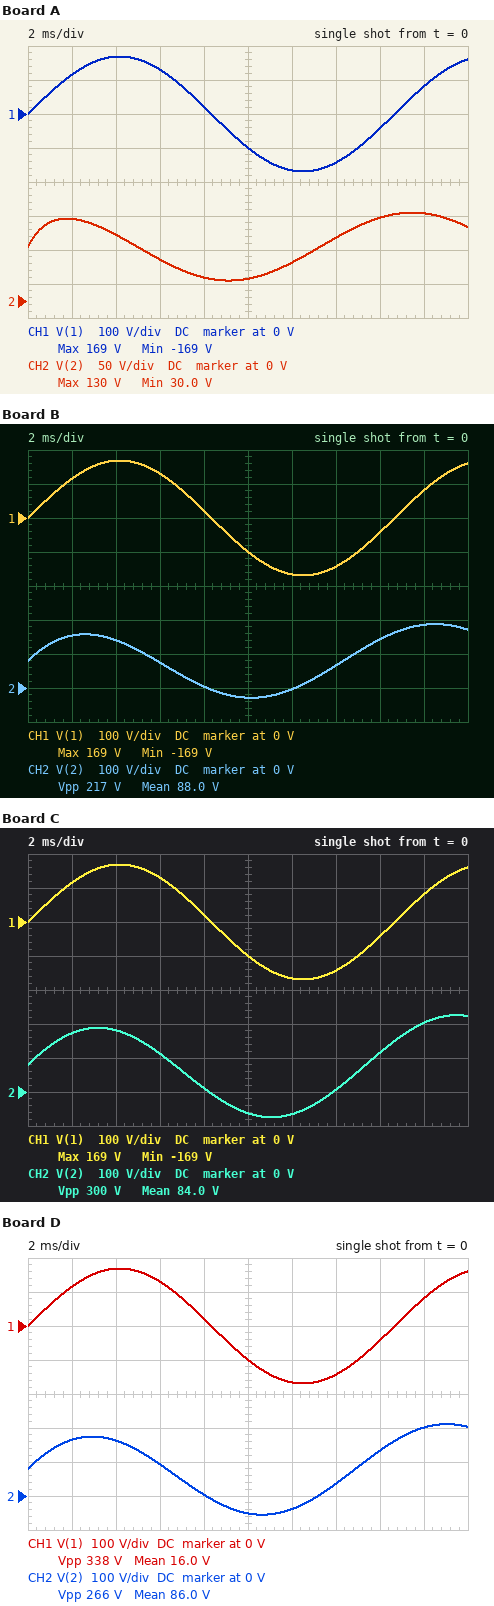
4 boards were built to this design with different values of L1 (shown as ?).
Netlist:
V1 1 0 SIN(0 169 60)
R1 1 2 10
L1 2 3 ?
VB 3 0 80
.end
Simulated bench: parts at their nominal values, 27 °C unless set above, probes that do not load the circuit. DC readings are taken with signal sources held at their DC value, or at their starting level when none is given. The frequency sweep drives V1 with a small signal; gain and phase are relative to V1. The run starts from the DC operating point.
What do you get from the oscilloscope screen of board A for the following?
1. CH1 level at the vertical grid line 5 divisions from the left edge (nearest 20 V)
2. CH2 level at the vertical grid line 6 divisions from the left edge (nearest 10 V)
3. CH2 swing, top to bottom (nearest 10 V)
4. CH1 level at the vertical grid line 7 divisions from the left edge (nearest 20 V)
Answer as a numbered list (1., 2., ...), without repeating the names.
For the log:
1. -100 V
2. 60 V
3. 100 V
4. -140 V
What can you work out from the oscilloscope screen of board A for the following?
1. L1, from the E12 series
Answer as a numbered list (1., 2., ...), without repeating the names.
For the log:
1. 8.2 mH
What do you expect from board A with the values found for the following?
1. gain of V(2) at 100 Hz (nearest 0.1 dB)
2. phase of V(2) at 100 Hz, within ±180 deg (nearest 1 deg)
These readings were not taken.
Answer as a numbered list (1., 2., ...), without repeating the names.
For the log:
1. -6.8 dB
2. 63 deg
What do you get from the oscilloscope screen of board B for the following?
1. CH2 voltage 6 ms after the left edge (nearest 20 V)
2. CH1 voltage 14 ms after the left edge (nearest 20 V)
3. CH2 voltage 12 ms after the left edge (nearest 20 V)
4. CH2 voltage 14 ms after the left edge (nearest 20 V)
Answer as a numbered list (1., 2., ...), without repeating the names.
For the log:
1. 80 V
2. -140 V
3. 0 V
4. 60 V
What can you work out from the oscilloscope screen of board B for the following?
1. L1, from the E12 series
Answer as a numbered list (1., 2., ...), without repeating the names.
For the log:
1. 22 mH
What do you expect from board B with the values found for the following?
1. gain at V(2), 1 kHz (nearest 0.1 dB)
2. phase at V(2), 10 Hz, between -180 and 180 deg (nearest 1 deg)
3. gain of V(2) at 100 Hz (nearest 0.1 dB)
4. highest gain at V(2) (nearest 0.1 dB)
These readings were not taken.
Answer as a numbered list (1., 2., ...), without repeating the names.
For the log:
1. 0 dB
2. 82 deg
3. -1.8 dB
4. 0 dB
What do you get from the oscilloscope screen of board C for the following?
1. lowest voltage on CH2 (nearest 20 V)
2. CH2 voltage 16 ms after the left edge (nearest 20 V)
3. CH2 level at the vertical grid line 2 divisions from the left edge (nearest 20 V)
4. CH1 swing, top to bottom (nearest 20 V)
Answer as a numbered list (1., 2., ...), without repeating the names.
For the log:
1. -80 V
2. 120 V
3. 180 V
4. 340 V
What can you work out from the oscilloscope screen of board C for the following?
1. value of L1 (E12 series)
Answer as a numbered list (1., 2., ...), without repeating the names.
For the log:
1. 47 mH
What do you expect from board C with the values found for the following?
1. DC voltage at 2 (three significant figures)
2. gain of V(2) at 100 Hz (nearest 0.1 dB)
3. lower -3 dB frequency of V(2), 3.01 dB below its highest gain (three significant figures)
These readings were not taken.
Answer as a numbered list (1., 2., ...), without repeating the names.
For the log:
1. 80.0 V
2. -0.5 dB
3. 33.9 Hz
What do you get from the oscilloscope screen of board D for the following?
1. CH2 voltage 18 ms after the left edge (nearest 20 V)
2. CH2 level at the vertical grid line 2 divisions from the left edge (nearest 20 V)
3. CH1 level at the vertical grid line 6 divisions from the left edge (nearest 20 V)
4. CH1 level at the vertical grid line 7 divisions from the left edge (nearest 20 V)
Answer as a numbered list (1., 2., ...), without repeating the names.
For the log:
1. 200 V
2. 160 V
3. -160 V
4. -140 V
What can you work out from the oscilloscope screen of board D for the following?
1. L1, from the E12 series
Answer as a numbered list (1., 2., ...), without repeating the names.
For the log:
1. 33 mH
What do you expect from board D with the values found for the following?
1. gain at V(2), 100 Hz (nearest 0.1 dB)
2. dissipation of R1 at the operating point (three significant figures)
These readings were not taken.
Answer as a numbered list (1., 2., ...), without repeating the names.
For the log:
1. -0.9 dB
2. 640 W
